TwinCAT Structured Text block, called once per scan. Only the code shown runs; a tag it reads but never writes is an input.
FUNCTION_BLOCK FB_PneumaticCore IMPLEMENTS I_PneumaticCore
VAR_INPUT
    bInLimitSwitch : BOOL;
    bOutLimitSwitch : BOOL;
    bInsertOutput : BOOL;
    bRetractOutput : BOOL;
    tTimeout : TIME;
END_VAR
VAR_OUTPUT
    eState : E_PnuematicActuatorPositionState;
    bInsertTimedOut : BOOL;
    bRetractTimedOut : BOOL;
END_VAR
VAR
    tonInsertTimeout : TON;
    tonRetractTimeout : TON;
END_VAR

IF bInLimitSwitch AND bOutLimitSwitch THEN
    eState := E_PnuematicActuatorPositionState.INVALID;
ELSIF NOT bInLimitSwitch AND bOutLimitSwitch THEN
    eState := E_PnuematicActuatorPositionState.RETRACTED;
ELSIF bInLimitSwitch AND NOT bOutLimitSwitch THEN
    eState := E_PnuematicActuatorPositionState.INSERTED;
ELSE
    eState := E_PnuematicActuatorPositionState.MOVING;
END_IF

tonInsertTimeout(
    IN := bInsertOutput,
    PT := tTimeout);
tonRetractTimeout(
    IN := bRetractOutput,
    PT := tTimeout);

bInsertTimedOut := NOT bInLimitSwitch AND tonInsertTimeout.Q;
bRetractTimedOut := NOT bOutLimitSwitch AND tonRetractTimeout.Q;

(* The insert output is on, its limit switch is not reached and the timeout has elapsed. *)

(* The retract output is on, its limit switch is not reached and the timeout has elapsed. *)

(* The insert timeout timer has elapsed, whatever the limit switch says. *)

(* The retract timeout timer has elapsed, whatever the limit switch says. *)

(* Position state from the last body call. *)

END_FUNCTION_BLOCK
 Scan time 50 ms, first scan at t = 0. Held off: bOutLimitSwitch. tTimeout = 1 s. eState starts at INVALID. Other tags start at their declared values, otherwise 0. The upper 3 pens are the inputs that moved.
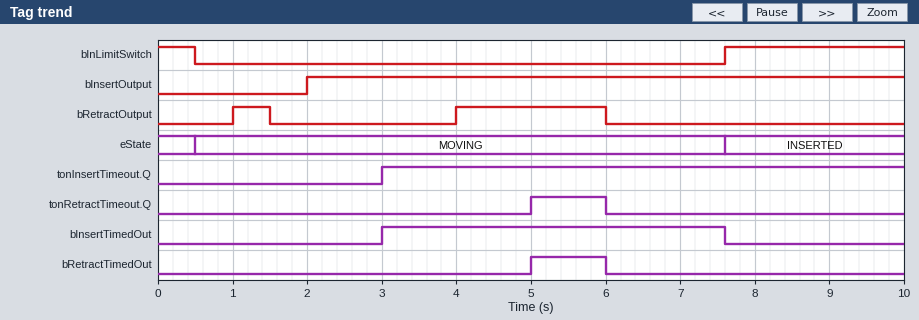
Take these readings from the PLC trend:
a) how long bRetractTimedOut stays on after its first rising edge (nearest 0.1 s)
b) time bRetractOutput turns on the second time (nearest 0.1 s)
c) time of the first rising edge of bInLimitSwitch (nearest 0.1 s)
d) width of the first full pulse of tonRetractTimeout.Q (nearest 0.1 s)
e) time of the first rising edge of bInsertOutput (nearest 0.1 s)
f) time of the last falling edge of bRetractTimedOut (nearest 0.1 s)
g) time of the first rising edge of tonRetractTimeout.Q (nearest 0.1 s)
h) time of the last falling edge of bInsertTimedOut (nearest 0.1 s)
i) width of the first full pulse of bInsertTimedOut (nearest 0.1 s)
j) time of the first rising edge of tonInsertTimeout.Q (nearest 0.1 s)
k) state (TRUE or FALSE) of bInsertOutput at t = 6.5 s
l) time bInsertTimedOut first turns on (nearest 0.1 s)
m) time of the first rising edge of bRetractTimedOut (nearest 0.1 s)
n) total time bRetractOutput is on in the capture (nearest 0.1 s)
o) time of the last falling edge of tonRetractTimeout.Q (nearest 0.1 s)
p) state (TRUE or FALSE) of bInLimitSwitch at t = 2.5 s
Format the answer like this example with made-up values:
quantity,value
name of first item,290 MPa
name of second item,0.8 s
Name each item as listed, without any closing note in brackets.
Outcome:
quantity,value
how long bRetractTimedOut stays on after its first rising edge,1.0 s
time bRetractOutput turns on the second time,4.0 s
time of the first rising edge of bInLimitSwitch,7.6 s
width of the first full pulse of tonRetractTimeout.Q,1.0 s
time of the first rising edge of bInsertOutput,2.0 s
time of the last falling edge of bRetractTimedOut,6.0 s
time of the first rising edge of tonRetractTimeout.Q,5.0 s
time of the last falling edge of bInsertTimedOut,7.6 s
width of the first full pulse of bInsertTimedOut,4.6 s
time of the first rising edge of tonInsertTimeout.Q,3.0 s
state (TRUE or FALSE) of bInsertOutput at t = 6.5 s,TRUE
time bInsertTimedOut first turns on,3.0 s
time of the first rising edge of bRetractTimedOut,5.0 s
total time bRetractOutput is on in the capture,2.5 s
time of the last falling edge of tonRetractTimeout.Q,6.0 s
state (TRUE or FALSE) of bInLimitSwitch at t = 2.5 s,FALSE
